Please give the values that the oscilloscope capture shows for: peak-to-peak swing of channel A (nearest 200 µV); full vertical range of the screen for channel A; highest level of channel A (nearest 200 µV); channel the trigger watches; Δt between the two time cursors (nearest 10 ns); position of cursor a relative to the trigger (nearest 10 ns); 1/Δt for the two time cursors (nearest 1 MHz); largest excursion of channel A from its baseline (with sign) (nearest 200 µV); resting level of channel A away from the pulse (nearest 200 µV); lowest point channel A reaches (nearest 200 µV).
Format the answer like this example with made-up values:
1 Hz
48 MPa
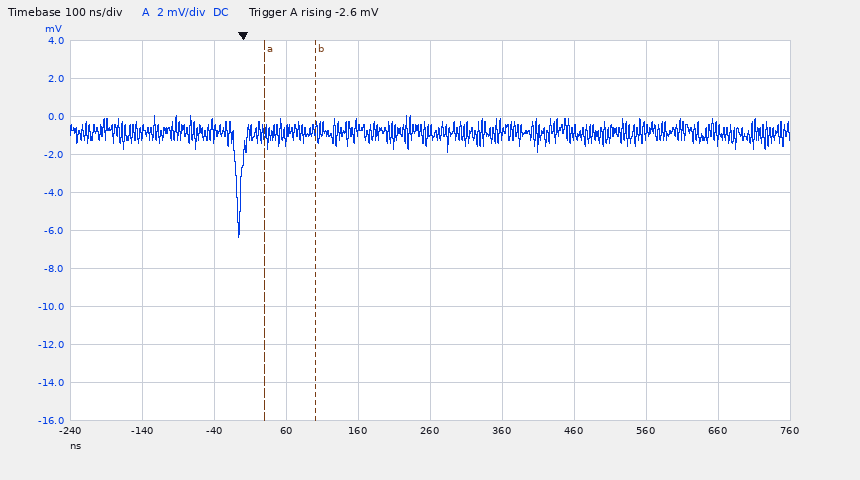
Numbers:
6.4 mV
20 mV
0.0 mV
channel A
70 ns
+30 ns
14 MHz
-5.6 mV
-800 µV
-6.4 mV
